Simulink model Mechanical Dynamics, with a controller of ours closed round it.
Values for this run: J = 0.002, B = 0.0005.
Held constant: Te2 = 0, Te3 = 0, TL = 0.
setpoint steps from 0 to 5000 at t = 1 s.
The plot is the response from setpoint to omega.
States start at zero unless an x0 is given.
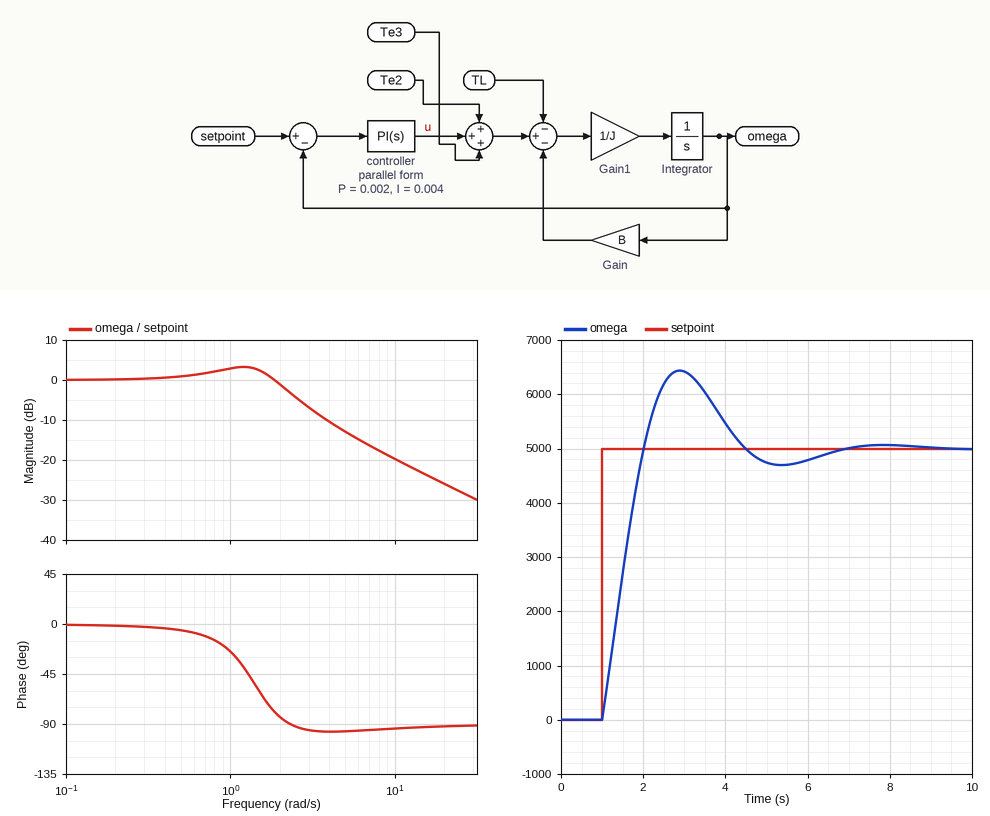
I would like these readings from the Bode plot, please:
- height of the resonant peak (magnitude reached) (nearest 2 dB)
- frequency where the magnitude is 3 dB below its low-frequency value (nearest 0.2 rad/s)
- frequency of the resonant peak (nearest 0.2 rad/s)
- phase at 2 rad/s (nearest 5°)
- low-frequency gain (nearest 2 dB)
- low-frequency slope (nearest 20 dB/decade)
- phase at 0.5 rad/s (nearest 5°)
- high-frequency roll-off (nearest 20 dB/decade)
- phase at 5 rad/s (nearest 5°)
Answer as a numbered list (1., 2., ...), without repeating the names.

1. 4 dB
2. 2.2 rad/s
3. 1.2 rad/s
4. -85°
5. 0 dB
6. 0 dB/decade
7. -5°
8. -20 dB/decade
9. -95°
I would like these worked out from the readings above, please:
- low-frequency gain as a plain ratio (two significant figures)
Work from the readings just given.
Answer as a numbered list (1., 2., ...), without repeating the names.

1. 1.0
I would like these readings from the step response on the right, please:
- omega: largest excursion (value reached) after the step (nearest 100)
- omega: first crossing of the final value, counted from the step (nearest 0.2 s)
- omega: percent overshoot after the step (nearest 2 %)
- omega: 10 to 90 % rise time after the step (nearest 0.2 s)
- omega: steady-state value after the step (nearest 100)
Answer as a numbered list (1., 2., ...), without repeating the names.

1. 6400
2. 1.0 s
3. 28 %
4. 0.8 s
5. 5000
